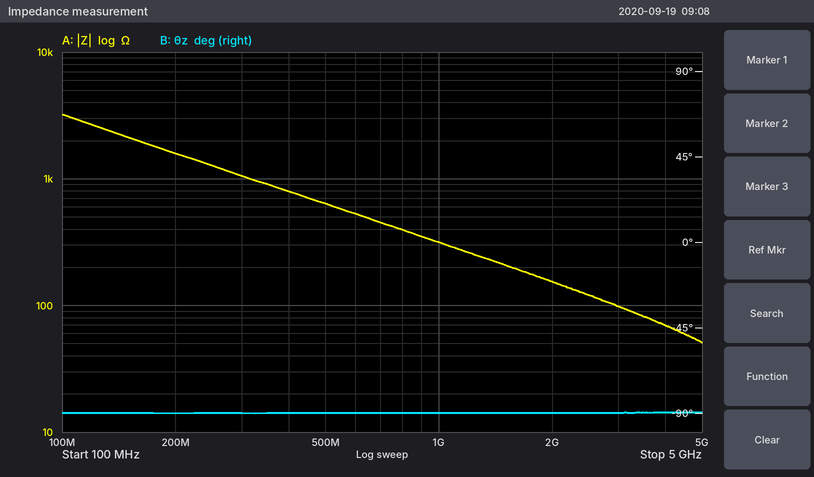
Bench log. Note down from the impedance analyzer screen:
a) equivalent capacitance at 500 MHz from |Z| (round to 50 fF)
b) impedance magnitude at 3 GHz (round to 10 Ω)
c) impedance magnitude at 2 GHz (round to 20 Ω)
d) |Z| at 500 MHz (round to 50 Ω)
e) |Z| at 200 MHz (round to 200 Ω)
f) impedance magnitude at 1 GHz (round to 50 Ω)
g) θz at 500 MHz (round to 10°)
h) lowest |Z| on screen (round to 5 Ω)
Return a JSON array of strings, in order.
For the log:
["500 fF", "100 Ω", "160 Ω", "650 Ω", "1.6 kΩ", "300 Ω", "-90°", "50 Ω"]
